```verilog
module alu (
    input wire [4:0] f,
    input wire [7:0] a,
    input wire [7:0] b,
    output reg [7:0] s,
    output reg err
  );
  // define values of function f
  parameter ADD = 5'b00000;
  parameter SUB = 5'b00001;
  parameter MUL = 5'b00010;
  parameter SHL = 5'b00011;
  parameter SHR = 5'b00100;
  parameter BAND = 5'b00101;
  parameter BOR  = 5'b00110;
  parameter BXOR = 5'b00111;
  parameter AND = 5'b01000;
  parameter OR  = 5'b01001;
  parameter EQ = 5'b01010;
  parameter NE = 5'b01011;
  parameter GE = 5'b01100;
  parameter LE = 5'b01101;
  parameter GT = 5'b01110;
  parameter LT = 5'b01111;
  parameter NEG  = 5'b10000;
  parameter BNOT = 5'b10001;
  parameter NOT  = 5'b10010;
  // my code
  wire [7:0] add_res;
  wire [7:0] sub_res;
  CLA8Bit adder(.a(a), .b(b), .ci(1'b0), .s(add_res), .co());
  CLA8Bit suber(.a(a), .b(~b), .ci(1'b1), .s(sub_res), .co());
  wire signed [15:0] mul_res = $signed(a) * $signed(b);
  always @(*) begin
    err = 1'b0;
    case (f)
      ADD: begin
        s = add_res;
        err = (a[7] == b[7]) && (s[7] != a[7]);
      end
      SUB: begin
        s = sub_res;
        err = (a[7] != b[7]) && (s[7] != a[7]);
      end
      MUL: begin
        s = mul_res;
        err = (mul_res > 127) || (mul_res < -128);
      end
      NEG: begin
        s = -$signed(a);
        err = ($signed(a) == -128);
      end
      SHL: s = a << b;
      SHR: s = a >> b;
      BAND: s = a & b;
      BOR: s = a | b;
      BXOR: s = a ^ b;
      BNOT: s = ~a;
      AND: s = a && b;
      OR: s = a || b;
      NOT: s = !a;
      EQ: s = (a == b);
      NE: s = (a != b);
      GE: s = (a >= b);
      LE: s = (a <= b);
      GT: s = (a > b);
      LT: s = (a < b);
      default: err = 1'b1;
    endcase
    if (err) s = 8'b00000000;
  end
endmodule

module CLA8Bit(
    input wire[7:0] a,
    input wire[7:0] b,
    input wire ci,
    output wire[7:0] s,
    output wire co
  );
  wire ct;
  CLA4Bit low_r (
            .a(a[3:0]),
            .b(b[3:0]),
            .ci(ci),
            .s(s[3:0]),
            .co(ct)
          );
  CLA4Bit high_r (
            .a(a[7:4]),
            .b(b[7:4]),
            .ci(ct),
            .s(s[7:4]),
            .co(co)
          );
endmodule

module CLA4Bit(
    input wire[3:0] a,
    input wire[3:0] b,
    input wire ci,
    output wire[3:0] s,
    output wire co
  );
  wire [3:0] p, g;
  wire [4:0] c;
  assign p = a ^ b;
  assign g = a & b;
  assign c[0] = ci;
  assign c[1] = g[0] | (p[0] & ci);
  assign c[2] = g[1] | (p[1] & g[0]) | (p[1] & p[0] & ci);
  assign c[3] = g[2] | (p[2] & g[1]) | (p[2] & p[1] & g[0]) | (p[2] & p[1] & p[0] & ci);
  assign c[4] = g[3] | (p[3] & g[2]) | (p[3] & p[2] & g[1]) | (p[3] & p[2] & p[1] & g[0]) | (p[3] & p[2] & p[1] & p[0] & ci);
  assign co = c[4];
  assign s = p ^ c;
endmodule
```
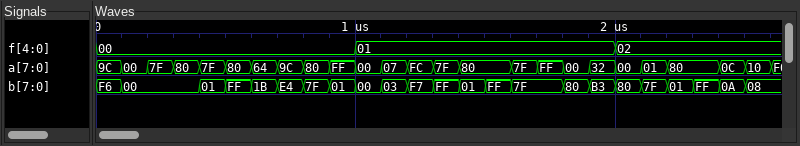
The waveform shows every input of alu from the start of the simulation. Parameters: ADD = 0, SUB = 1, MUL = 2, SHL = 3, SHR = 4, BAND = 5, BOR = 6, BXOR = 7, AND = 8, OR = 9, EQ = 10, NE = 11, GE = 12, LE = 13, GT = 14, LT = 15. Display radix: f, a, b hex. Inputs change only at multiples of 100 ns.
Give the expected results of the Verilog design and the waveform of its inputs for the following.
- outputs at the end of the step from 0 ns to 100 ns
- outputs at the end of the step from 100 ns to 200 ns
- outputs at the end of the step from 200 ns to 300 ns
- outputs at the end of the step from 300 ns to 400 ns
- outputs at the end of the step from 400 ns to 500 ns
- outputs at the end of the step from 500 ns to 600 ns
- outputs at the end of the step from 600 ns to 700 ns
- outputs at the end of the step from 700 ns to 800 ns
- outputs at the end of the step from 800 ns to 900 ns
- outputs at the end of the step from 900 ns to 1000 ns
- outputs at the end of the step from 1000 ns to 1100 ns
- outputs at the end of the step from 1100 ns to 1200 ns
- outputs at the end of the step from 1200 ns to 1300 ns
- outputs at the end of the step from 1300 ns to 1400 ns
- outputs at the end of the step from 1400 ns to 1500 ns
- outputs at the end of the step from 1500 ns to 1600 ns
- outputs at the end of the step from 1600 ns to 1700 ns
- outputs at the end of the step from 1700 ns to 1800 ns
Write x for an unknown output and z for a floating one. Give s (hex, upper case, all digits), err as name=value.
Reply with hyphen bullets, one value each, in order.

- s=92, err=0
- s=00, err=0
- s=7F, err=0
- s=80, err=0
- s=00, err=1
- s=00, err=1
- s=7F, err=0
- s=80, err=0
- s=FF, err=0
- s=00, err=0
- s=00, err=0
- s=04, err=0
- s=05, err=0
- s=00, err=1
- s=00, err=1
- s=81, err=0
- s=00, err=0
- s=80, err=0
